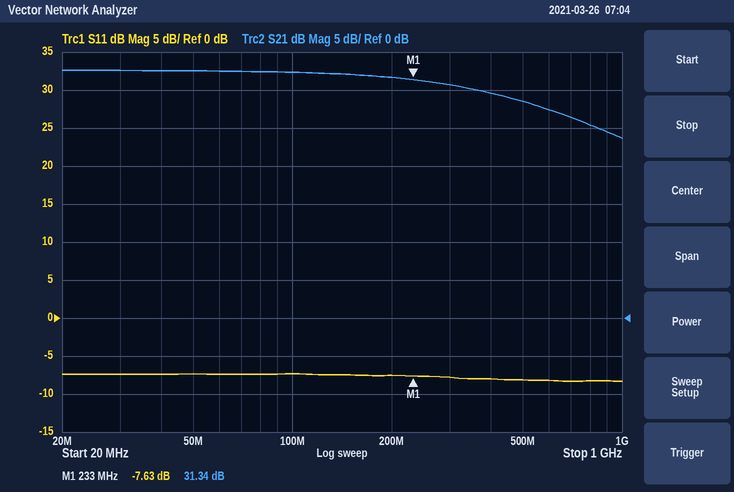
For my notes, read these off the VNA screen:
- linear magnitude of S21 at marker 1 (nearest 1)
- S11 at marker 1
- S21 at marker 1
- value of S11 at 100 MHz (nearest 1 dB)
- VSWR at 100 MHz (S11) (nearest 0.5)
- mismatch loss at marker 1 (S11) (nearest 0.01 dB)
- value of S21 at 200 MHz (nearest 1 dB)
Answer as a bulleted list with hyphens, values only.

- 37
- -7.63 dB
- 31.34 dB
- -7 dB
- 2.5
- 0.82 dB
- 32 dB
